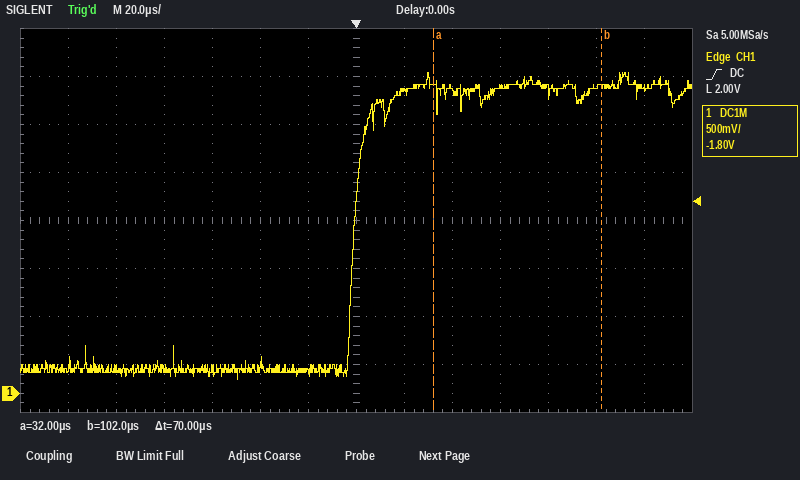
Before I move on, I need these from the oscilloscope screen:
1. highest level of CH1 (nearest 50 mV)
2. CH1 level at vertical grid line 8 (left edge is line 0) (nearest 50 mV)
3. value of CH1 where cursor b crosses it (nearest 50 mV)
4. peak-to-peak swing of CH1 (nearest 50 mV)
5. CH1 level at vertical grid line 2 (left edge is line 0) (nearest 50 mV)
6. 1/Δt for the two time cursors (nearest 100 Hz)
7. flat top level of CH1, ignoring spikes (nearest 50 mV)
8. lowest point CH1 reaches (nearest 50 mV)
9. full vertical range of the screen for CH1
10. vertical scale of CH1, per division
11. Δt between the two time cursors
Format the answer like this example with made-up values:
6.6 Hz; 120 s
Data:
3.35 V; 3.15 V; 3.20 V; 3.20 V; 250 mV; 14.3 kHz; 3.20 V; 150 mV; 4 V; 500 mV; 70 µs
